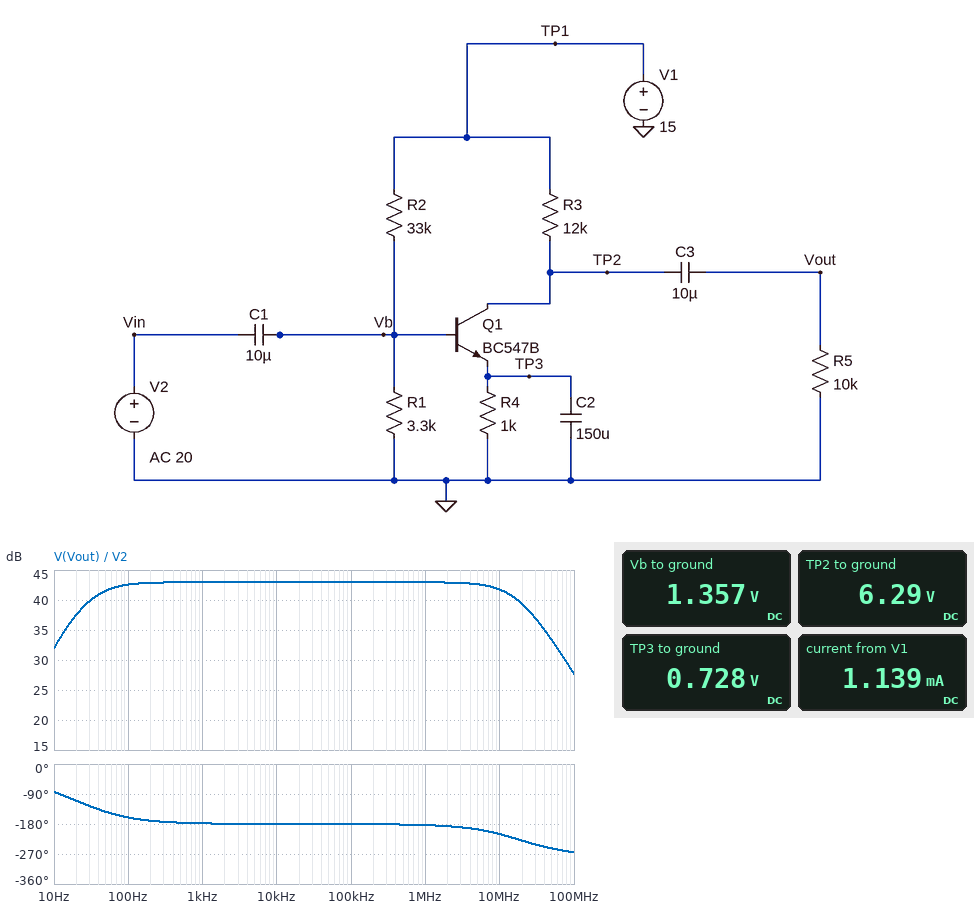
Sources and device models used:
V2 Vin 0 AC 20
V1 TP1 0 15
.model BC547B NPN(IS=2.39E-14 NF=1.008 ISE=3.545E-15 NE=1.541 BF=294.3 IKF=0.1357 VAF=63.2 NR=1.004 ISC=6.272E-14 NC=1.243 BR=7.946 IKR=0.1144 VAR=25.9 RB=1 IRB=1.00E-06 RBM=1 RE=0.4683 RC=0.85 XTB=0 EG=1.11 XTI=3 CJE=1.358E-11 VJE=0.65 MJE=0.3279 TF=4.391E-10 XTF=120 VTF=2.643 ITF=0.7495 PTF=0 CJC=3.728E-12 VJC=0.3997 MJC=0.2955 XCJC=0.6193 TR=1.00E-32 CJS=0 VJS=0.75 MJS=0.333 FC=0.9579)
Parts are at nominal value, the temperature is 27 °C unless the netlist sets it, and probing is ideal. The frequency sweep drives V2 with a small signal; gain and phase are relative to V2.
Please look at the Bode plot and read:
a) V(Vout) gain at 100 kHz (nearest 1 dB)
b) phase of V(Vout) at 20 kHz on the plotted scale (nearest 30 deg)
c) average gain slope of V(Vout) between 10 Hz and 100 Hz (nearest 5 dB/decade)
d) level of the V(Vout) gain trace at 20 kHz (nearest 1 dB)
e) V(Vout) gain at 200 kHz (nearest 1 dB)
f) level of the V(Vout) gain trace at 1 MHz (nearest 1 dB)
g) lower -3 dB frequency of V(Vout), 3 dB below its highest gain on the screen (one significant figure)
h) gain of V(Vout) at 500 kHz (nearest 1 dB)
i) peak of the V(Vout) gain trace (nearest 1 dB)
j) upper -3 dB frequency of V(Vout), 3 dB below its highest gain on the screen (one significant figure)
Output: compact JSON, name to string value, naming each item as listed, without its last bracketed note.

{"V(Vout) gain at 100 kHz": "43 dB", "phase of V(Vout) at 20 kHz on the plotted scale": "-180 deg", "average gain slope of V(Vout) between 10 Hz and 100 Hz": "10 dB/decade", "level of the V(Vout) gain trace at 20 kHz": "43 dB", "V(Vout) gain at 200 kHz": "43 dB", "level of the V(Vout) gain trace at 1 MHz": "43 dB", "lower -3 dB frequency of V(Vout), 3 dB below its highest gain on the screen": "30 Hz", "gain of V(Vout) at 500 kHz": "43 dB", "peak of the V(Vout) gain trace": "43 dB", "upper -3 dB frequency of V(Vout), 3 dB below its highest gain on the screen": "20 MHz"}
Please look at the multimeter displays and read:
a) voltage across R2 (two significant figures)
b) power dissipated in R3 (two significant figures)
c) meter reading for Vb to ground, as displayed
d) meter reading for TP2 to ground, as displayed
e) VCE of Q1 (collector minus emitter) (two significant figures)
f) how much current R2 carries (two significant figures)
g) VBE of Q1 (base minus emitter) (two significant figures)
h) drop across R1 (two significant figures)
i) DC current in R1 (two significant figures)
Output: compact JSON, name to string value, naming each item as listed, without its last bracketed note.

{"voltage across R2": "14 V", "power dissipated in R3": "6.3 mW", "meter reading for Vb to ground, as displayed": "1.357 V", "meter reading for TP2 to ground, as displayed": "6.29 V", "VCE of Q1 (collector minus emitter)": "5.6 V", "how much current R2 carries": "410 µA", "VBE of Q1 (base minus emitter)": "630 mV", "drop across R1": "1.4 V", "DC current in R1": "410 µA"}
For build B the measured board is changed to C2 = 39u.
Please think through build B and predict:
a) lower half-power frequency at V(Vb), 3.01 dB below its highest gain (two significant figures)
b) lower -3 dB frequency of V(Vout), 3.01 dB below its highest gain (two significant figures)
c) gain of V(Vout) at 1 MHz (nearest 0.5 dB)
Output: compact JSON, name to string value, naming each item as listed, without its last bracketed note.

{"lower half-power frequency at V(Vb), 3.01 dB below its highest gain": "5.4 Hz", "lower -3 dB frequency of V(Vout), 3.01 dB below its highest gain": "110 Hz", "gain of V(Vout) at 1 MHz": "43.0 dB"}
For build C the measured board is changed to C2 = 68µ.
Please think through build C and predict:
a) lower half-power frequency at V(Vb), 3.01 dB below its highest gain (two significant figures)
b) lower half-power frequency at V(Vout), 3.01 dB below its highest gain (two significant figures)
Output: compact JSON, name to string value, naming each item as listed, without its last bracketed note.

{"lower half-power frequency at V(Vb), 3.01 dB below its highest gain": "5.5 Hz", "lower half-power frequency at V(Vout), 3.01 dB below its highest gain": "65 Hz"}
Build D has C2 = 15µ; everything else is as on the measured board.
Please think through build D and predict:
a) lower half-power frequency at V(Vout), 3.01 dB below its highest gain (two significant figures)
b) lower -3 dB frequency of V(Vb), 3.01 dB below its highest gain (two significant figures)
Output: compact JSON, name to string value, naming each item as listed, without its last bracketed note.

{"lower half-power frequency at V(Vout), 3.01 dB below its highest gain": "290 Hz", "lower -3 dB frequency of V(Vb), 3.01 dB below its highest gain": "5.4 Hz"}
